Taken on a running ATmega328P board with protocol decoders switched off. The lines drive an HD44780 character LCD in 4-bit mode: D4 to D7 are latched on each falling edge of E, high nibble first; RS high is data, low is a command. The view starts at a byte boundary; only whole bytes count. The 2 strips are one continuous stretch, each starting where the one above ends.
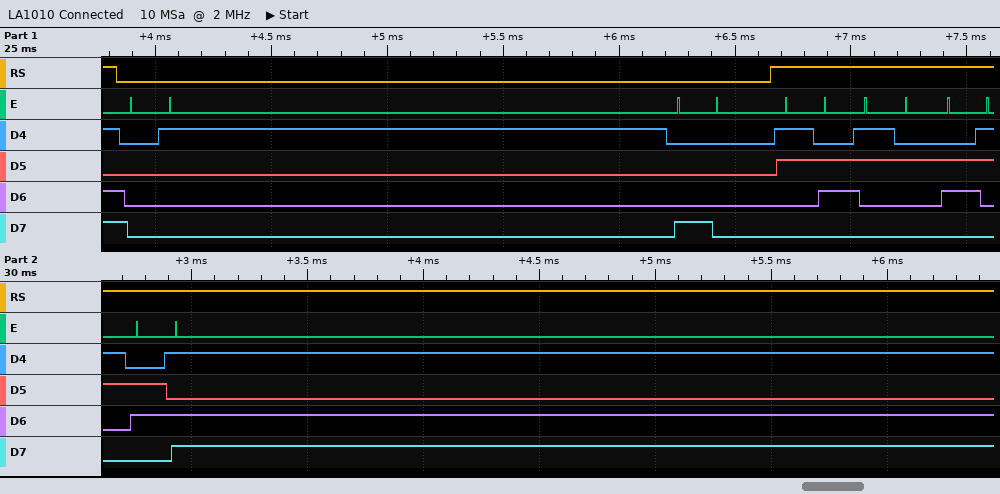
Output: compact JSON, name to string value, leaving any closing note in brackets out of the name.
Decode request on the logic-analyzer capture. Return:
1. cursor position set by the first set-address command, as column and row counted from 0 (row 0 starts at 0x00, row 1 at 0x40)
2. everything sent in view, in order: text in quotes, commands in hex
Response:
{"cursor position set by the first set-address command, as column and row counted from 0": "column 0, row 0", "everything sent in view, in order: text in quotes, commands in hex": "0x01 0x80 \"62cm\""}
